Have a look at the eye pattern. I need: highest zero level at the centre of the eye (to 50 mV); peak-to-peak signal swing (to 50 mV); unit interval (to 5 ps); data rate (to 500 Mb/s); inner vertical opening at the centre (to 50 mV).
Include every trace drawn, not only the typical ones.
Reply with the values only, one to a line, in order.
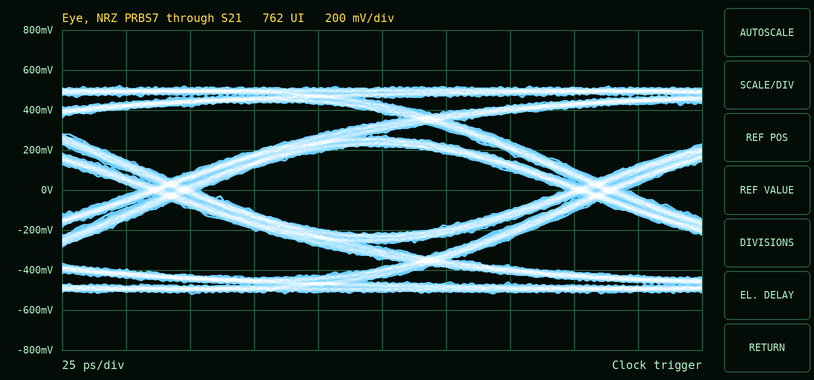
-200 mV
1.05 V
165 ps
6.0 Gb/s
450 mV
